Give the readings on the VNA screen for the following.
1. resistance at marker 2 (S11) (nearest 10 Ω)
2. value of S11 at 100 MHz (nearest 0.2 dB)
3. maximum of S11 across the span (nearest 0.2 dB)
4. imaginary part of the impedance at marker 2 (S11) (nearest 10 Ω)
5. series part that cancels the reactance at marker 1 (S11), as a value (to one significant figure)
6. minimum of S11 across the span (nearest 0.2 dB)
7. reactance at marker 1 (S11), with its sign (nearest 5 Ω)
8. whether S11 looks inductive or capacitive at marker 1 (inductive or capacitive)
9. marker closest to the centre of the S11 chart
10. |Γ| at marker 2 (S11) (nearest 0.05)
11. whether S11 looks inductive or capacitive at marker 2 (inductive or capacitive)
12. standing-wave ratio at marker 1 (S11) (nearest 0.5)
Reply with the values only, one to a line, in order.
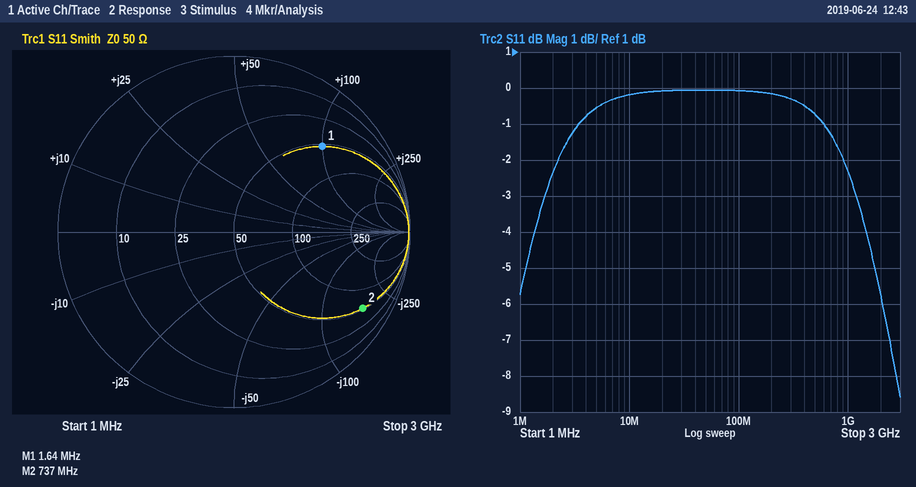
50 Ω
0.0 dB
0.0 dB
-170 Ω
1.0 nF
-8.6 dB
+100 Ω
inductive
marker 1
0.85
capacitive
5.5
